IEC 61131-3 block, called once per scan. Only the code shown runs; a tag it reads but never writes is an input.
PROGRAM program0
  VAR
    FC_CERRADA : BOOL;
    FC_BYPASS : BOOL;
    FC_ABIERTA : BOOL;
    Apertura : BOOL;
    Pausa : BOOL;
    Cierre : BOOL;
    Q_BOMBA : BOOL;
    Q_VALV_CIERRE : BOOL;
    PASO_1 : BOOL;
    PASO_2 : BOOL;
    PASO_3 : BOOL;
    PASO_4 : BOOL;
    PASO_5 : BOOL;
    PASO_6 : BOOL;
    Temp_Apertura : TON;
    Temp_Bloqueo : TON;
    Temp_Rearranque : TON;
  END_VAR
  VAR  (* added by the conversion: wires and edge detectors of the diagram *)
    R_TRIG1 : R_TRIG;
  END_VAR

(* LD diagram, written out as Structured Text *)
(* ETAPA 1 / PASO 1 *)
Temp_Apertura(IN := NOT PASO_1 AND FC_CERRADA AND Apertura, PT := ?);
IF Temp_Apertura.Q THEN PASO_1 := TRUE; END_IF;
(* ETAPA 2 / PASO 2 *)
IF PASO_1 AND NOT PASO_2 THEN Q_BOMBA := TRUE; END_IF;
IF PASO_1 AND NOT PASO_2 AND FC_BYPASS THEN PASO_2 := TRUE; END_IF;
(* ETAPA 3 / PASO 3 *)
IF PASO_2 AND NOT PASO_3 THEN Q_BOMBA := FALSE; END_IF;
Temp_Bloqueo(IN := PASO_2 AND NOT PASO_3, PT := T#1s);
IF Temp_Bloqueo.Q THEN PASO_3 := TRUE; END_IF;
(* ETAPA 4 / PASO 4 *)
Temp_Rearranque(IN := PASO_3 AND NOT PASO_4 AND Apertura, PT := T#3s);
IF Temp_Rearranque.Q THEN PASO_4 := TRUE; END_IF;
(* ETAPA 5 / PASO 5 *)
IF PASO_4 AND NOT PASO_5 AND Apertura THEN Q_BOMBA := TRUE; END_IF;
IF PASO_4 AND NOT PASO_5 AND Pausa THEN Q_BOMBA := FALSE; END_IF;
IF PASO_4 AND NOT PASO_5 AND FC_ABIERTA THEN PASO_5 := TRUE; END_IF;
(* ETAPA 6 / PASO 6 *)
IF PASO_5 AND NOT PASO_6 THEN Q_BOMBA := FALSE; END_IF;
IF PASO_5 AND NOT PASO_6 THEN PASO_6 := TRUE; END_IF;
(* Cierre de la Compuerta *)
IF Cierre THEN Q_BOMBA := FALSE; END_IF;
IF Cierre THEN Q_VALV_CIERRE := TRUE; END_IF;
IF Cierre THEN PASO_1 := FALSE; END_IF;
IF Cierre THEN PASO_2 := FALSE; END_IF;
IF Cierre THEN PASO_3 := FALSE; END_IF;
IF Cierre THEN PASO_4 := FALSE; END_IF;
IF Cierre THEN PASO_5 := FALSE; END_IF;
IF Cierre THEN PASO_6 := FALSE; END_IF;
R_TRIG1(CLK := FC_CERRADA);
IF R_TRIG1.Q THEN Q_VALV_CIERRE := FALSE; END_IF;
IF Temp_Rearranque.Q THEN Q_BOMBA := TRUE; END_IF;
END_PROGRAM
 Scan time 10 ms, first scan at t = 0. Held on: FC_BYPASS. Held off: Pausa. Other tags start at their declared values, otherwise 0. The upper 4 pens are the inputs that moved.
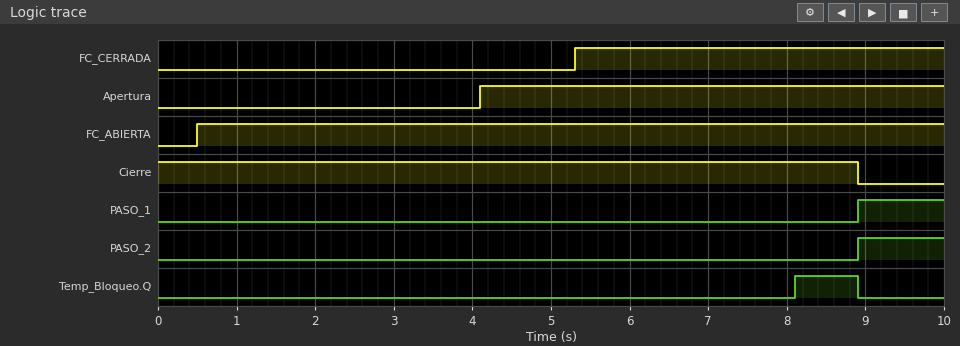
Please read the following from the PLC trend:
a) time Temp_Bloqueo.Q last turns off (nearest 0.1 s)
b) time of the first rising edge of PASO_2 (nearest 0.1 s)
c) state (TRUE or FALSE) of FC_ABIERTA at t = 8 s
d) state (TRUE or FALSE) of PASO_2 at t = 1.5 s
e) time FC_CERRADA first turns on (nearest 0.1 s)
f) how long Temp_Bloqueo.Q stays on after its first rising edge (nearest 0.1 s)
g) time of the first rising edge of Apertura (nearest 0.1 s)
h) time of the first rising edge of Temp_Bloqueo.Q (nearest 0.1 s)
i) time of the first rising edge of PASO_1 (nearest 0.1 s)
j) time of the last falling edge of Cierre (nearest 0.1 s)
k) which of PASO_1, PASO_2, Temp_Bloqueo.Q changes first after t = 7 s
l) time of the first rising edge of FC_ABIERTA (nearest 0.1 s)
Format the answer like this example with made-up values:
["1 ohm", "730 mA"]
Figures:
["8.9 s", "8.9 s", "TRUE", "FALSE", "5.3 s", "0.8 s", "4.1 s", "8.1 s", "8.9 s", "8.9 s", "Temp_Bloqueo.Q", "0.5 s"]
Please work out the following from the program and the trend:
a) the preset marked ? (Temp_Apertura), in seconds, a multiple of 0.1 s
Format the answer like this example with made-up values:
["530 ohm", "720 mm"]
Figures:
["1.8 s"]
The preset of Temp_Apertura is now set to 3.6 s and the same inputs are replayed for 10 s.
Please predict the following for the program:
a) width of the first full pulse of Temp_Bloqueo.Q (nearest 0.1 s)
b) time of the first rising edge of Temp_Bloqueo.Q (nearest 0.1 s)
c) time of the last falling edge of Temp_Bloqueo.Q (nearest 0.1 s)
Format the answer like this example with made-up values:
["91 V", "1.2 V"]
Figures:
["0.0 s", "9.9 s", "9.9 s"]
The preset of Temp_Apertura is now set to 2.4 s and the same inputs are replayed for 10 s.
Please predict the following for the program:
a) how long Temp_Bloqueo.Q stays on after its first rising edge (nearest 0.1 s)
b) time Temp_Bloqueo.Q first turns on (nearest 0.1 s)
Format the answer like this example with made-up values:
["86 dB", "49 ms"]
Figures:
["0.2 s", "8.7 s"]
